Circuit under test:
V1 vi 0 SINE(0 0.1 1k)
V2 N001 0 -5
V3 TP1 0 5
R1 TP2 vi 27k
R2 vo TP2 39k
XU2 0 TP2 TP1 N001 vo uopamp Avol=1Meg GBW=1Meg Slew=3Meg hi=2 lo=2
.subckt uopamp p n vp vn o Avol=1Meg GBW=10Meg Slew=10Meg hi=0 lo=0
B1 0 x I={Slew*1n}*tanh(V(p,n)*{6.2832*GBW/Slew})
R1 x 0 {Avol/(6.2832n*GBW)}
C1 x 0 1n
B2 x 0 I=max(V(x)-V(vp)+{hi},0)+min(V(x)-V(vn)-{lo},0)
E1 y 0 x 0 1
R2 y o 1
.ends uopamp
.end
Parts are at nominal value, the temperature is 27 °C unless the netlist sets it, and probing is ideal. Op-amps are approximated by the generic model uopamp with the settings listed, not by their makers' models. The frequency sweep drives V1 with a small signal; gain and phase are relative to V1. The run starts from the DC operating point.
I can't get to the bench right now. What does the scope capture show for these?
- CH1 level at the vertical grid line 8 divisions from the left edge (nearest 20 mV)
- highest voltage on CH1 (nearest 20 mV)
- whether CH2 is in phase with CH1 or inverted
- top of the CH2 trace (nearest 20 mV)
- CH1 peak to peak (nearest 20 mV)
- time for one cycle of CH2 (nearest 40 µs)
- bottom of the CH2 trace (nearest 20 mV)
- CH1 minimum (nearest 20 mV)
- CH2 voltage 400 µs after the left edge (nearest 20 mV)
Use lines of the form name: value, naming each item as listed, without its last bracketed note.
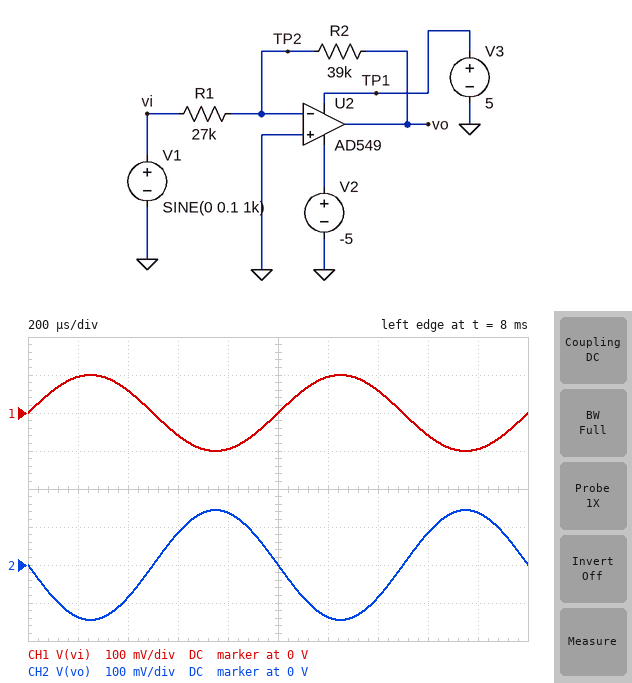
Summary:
CH1 level at the vertical grid line 8 divisions from the left edge: -60 mV
highest voltage on CH1: 100 mV
whether CH2 is in phase with CH1 or inverted: inverted
top of the CH2 trace: 140 mV
CH1 peak to peak: 200 mV
time for one cycle of CH2: 1.00 ms
bottom of the CH2 trace: -140 mV
CH1 minimum: -100 mV
CH2 voltage 400 µs after the left edge: -80 mV
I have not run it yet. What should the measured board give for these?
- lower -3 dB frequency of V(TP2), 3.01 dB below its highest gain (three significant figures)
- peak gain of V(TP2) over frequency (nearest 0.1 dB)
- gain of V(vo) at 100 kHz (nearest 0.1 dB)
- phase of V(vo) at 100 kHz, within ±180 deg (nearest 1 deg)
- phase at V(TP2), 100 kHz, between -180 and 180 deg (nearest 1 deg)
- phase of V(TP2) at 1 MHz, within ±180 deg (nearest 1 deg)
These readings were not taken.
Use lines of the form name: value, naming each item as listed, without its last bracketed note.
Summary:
lower -3 dB frequency of V(TP2), 3.01 dB below its highest gain: 409 kHz
peak gain of V(TP2) over frequency: -4.6 dB
gain of V(vo) at 100 kHz: 2.9 dB
phase of V(vo) at 100 kHz, within ±180 deg: 166 deg
phase at V(TP2), 100 kHz, between -180 and 180 deg: 76 deg
phase of V(TP2) at 1 MHz, within ±180 deg: 22 deg
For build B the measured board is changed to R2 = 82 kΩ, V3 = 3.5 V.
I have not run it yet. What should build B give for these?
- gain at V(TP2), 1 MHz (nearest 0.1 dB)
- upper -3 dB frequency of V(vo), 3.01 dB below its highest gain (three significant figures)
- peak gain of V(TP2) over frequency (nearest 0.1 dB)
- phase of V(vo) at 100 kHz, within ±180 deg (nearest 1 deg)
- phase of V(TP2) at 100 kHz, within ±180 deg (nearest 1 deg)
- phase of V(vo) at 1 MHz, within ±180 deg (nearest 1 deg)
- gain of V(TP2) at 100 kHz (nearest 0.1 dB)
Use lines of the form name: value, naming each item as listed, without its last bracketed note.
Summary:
gain at V(TP2), 1 MHz: -2.7 dB
upper -3 dB frequency of V(vo), 3.01 dB below its highest gain: 248 kHz
peak gain of V(TP2) over frequency: -2.5 dB
phase of V(vo) at 100 kHz, within ±180 deg: 158 deg
phase of V(TP2) at 100 kHz, within ±180 deg: 68 deg
phase of V(vo) at 1 MHz, within ±180 deg: 104 deg
gain of V(TP2) at 100 kHz: -11.0 dB
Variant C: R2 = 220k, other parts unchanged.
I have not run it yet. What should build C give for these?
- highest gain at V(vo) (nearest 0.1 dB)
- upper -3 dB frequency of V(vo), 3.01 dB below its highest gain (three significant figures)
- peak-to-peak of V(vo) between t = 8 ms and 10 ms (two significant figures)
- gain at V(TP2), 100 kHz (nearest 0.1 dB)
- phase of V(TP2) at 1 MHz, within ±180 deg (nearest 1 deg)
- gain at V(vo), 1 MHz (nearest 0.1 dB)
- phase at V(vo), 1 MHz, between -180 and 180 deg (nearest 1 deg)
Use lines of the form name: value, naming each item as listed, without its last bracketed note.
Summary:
highest gain at V(vo): 18.2 dB
upper -3 dB frequency of V(vo), 3.01 dB below its highest gain: 109 kHz
peak-to-peak of V(vo) between t = 8 ms and 10 ms: 1.6 V
gain at V(TP2), 100 kHz: -4.4 dB
phase of V(TP2) at 1 MHz, within ±180 deg: 6 deg
gain at V(vo), 1 MHz: -1.1 dB
phase at V(vo), 1 MHz, between -180 and 180 deg: 96 deg
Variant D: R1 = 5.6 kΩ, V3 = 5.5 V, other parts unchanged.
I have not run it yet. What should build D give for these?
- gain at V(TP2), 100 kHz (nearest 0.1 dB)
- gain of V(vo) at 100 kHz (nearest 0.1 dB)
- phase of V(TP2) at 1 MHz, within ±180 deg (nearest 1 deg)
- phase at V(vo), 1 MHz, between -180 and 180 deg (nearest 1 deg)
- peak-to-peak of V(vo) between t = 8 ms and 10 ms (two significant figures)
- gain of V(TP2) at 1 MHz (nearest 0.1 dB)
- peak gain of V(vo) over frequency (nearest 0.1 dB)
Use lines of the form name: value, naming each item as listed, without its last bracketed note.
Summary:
gain at V(TP2), 100 kHz: -5.3 dB
gain of V(vo) at 100 kHz: 14.7 dB
phase of V(TP2) at 1 MHz, within ±180 deg: 7 deg
phase at V(vo), 1 MHz, between -180 and 180 deg: 97 deg
peak-to-peak of V(vo) between t = 8 ms and 10 ms: 1.4 V
gain of V(TP2) at 1 MHz: -1.2 dB
peak gain of V(vo) over frequency: 16.9 dB
